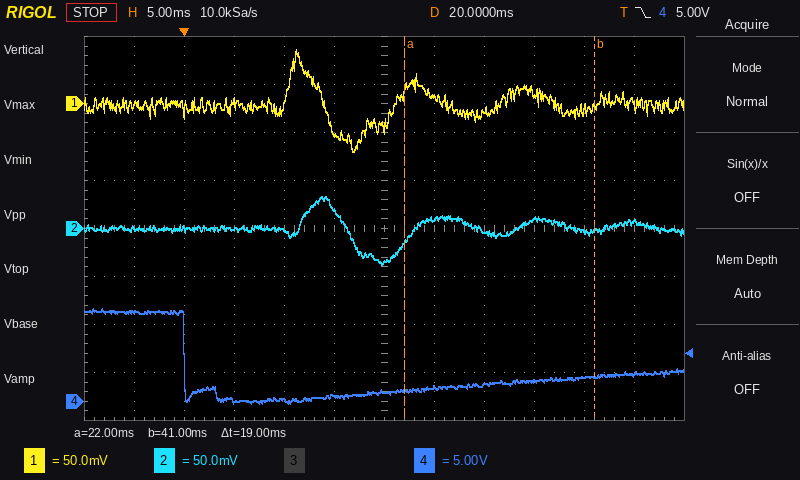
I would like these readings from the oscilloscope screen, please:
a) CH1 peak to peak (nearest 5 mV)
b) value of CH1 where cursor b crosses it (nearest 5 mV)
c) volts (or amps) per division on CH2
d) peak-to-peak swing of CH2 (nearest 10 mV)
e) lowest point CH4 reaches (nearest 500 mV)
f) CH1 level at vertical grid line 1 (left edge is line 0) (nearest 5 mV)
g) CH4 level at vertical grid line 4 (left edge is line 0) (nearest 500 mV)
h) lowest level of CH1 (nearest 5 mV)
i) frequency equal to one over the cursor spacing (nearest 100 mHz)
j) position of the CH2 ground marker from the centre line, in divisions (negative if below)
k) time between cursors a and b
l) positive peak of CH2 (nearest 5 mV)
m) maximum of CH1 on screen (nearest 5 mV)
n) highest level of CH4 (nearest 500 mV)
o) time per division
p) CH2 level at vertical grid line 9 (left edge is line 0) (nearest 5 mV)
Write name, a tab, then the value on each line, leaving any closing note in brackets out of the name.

CH1 peak to peak	105 mV
value of CH1 where cursor b crosses it	-5 mV
volts (or amps) per division on CH2	50 mV
peak-to-peak swing of CH2	70 mV
lowest point CH4 reaches	0.0 V
CH1 level at vertical grid line 1 (left edge is line 0)	0 mV
CH4 level at vertical grid line 4 (left edge is line 0)	0.0 V
lowest level of CH1	-50 mV
frequency equal to one over the cursor spacing	52.6 Hz
position of the CH2 ground marker from the centre line, in divisions	0.0 div
time between cursors a and b	19 ms
positive peak of CH2	35 mV
maximum of CH1 on screen	55 mV
highest level of CH4	9.5 V
time per division	5 ms
CH2 level at vertical grid line 9 (left edge is line 0)	10 mV
